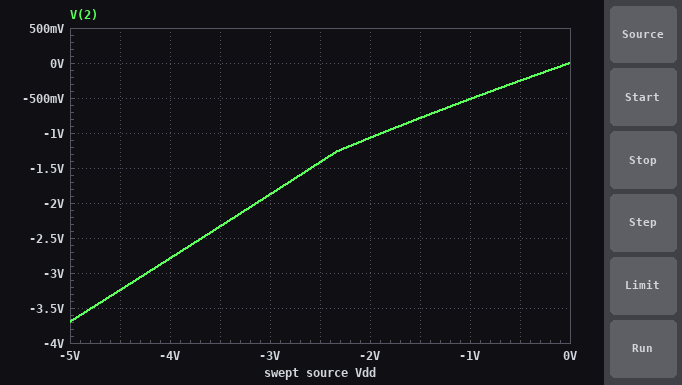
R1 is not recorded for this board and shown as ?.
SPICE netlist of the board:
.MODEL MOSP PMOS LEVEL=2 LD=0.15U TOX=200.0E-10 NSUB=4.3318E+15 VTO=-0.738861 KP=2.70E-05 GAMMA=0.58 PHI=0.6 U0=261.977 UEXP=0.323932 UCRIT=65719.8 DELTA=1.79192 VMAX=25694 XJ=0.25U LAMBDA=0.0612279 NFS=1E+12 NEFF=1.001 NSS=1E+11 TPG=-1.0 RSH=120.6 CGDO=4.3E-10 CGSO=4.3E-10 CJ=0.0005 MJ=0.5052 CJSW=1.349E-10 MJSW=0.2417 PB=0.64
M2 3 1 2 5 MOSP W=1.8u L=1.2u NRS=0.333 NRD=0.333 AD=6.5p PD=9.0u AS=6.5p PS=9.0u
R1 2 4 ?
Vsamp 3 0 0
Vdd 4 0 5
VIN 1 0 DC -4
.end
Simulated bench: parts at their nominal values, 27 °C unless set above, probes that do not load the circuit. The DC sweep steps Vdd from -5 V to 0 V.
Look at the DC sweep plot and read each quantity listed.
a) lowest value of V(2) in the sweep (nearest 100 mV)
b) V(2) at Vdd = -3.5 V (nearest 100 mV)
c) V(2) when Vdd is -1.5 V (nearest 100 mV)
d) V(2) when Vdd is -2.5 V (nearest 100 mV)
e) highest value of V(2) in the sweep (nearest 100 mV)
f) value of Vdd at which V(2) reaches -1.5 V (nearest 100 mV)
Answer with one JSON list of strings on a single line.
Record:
["-3.7 V", "-2.3 V", "-800 mV", "-1.4 V", "0 V", "-2.6 V"]
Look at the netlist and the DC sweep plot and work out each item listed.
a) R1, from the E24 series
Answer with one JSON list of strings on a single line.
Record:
["11 kΩ"]
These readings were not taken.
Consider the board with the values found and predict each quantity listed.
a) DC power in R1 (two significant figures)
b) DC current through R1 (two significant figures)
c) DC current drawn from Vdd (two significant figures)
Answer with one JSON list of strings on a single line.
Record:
["550 µW", "220 µA", "220 µA"]
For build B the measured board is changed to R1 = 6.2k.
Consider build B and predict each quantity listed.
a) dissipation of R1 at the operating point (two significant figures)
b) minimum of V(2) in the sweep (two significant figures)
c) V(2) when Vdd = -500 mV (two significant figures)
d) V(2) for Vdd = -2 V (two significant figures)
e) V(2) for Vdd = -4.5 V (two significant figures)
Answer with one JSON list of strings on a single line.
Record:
["470 µW", "-4.2 V", "-320 mV", "-1.4 V", "-3.8 V"]
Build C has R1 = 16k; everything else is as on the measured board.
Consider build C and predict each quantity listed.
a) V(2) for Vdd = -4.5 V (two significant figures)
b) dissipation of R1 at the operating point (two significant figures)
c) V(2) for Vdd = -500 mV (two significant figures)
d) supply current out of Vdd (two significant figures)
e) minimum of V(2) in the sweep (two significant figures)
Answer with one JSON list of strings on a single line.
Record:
["-2.7 V", "570 µW", "-210 mV", "190 µA", "-3.2 V"]
